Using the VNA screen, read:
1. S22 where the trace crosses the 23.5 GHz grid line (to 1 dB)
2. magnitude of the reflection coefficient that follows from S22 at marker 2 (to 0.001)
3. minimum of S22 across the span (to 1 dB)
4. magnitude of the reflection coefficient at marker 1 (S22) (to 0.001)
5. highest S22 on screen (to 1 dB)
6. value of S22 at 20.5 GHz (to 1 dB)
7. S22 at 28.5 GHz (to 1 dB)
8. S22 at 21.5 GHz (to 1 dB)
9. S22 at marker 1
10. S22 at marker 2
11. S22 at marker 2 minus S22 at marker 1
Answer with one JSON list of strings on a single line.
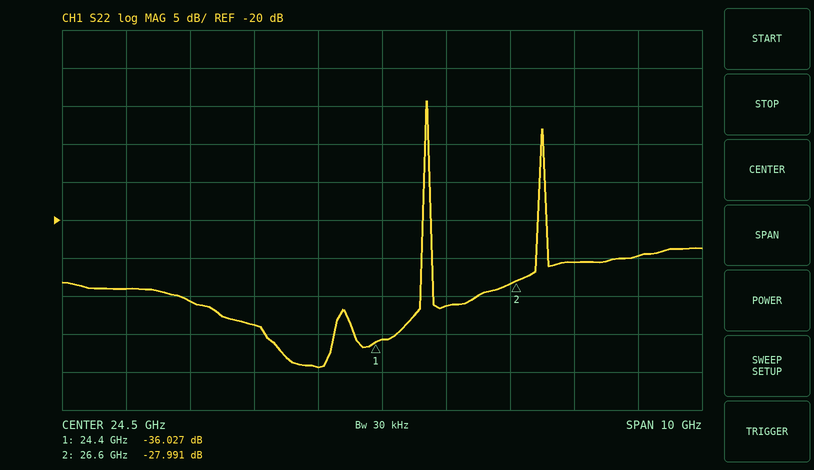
["-39 dB", "0.040", "-39 dB", "0.016", "-4 dB", "-29 dB", "-25 dB", "-31 dB", "-36.027 dB", "-27.991 dB", "8.036 dB"]
